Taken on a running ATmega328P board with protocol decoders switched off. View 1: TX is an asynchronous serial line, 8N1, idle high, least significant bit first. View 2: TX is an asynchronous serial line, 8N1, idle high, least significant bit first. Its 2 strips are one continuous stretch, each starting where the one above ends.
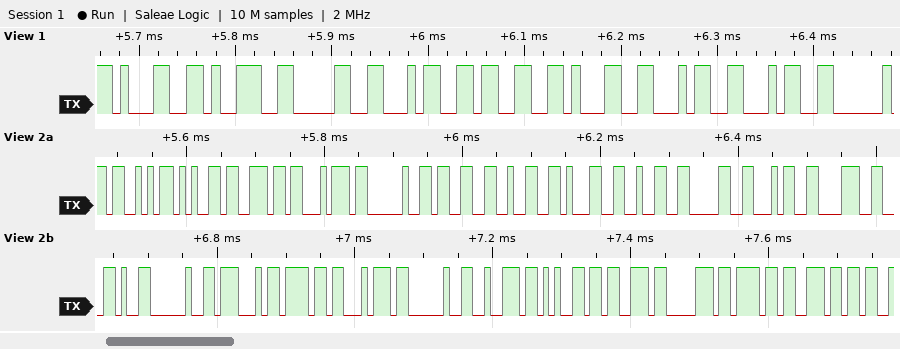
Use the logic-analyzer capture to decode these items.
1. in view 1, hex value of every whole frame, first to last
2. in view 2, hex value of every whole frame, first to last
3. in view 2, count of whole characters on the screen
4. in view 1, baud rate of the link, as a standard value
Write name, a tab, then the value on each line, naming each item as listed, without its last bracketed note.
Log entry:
in view 1, hex value of every whole frame, first to last	31 39 30 34 33 31 34 34
in view 2, hex value of every whole frame, first to last	53 65 6E 74 20 33 32 31 32 30 34 38 2C 20 47 6F 74 20 72 65 73 70 6F 6E
in view 2, count of whole characters on the screen	24
in view 1, baud rate of the link, as a standard value	115200 baud
